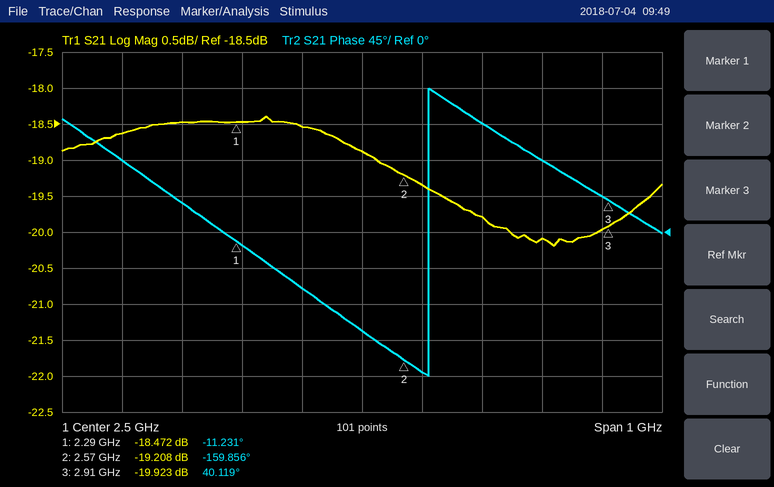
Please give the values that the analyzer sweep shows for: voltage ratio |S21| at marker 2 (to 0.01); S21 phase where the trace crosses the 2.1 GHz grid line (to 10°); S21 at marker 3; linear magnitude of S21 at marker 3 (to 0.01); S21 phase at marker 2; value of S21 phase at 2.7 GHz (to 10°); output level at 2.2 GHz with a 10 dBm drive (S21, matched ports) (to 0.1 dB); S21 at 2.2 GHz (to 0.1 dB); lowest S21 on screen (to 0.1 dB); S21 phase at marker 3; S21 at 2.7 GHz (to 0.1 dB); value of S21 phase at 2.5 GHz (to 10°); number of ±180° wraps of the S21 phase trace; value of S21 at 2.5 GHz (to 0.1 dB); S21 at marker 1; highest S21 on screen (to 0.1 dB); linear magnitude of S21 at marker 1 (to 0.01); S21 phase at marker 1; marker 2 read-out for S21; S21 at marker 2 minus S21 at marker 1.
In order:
0.11
90°
-19.923 dB
0.10
-159.856°
140°
-8.5 dBm
-18.5 dB
-20.2 dB
40.119°
-19.8 dB
-120°
1
-18.9 dB
-18.472 dB
-18.4 dB
0.12
-11.231°
-19.208 dB
-0.736 dB
